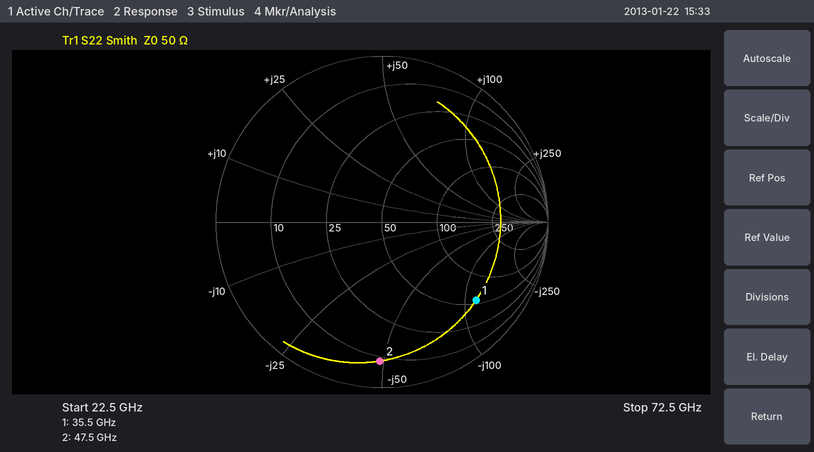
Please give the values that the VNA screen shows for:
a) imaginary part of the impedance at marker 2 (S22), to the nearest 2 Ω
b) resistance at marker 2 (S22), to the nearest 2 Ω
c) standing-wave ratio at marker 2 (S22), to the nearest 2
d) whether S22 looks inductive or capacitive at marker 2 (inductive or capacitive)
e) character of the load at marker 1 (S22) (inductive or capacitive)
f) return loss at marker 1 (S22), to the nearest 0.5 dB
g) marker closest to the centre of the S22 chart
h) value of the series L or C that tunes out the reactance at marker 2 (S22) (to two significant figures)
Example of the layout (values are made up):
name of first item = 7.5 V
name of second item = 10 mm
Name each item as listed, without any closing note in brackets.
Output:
imaginary part of the impedance at marker 2 (S22), to the nearest 2 Ω = -48 Ω
resistance at marker 2 (S22), to the nearest 2 Ω = 8 Ω
standing-wave ratio at marker 2 (S22), to the nearest 2 = 12
whether S22 looks inductive or capacitive at marker 2 = capacitive
character of the load at marker 1 (S22) = capacitive
return loss at marker 1 (S22), to the nearest 0.5 dB = 2.5 dB
marker closest to the centre of the S22 chart = marker 1
value of the series L or C that tunes out the reactance at marker 2 (S22) = 160 pH
